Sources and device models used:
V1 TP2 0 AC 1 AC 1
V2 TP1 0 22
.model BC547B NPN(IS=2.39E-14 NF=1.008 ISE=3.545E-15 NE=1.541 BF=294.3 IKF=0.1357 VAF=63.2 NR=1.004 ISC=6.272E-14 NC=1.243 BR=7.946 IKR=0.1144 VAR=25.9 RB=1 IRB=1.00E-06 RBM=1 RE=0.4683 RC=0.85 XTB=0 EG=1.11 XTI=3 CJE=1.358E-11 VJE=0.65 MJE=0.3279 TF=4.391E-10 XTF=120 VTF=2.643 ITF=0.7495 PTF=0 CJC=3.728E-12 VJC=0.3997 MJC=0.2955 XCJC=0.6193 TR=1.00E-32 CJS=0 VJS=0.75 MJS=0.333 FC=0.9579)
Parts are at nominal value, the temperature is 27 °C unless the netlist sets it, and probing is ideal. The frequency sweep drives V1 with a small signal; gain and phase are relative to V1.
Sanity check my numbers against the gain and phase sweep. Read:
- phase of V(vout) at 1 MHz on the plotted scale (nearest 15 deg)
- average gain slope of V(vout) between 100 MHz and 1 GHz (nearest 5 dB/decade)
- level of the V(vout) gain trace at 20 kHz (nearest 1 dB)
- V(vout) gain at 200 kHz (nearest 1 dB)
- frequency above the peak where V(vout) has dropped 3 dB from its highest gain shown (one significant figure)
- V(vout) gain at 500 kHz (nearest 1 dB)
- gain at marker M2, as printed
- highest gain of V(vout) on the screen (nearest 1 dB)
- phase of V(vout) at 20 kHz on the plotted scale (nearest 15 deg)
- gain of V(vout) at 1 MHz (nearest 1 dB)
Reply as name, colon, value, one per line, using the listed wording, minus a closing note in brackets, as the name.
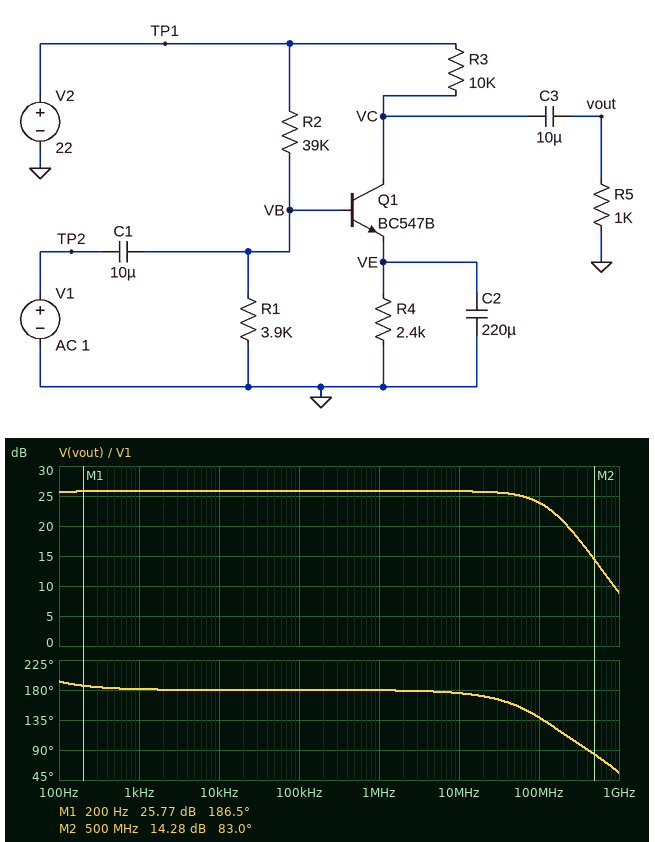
phase of V(vout) at 1 MHz on the plotted scale: 180 deg
average gain slope of V(vout) between 100 MHz and 1 GHz: -15 dB/decade
level of the V(vout) gain trace at 20 kHz: 26 dB
V(vout) gain at 200 kHz: 26 dB
frequency above the peak where V(vout) has dropped 3 dB from its highest gain shown: 100 MHz
V(vout) gain at 500 kHz: 26 dB
gain at marker M2, as printed: 14.28 dB
highest gain of V(vout) on the screen: 26 dB
phase of V(vout) at 20 kHz on the plotted scale: 180 deg
gain of V(vout) at 1 MHz: 26 dB
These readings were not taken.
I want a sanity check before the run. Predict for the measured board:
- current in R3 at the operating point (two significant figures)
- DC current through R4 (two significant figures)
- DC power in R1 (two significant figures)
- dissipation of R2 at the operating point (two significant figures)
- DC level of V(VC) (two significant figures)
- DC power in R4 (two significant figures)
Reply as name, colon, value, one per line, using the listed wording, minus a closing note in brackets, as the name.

current in R3 at the operating point: 570 µA
DC current through R4: 570 µA
DC power in R1: 1.0 mW
dissipation of R2 at the operating point: 10 mW
DC level of V(VC): 16 V
DC power in R4: 790 µW
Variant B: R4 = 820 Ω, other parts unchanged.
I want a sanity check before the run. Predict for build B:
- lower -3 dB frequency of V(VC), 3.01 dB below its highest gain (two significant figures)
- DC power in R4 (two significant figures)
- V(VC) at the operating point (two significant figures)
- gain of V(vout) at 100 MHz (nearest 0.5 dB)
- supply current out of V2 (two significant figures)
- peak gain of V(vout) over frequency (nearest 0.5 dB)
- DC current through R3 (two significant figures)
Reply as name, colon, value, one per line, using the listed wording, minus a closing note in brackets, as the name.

lower -3 dB frequency of V(VC), 3.01 dB below its highest gain: 42 Hz
DC power in R4: 2.2 mW
V(VC) at the operating point: 5.8 V
gain of V(vout) at 100 MHz: 31.0 dB
supply current out of V2: 2.1 mA
peak gain of V(vout) over frequency: 34.5 dB
DC current through R3: 1.6 mA
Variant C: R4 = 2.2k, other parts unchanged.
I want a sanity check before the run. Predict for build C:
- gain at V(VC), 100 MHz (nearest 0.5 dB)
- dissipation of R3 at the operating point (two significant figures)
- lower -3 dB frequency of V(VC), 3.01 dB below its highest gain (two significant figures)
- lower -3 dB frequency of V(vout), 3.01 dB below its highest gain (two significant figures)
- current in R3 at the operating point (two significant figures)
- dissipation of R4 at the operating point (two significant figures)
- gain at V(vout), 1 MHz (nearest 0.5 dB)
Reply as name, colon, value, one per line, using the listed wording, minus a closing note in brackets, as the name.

gain at V(VC), 100 MHz: 24.5 dB
dissipation of R3 at the operating point: 3.9 mW
lower -3 dB frequency of V(VC), 3.01 dB below its highest gain: 6.4 Hz
lower -3 dB frequency of V(vout), 3.01 dB below its highest gain: 20 Hz
current in R3 at the operating point: 620 µA
dissipation of R4 at the operating point: 860 µW
gain at V(vout), 1 MHz: 26.5 dB
